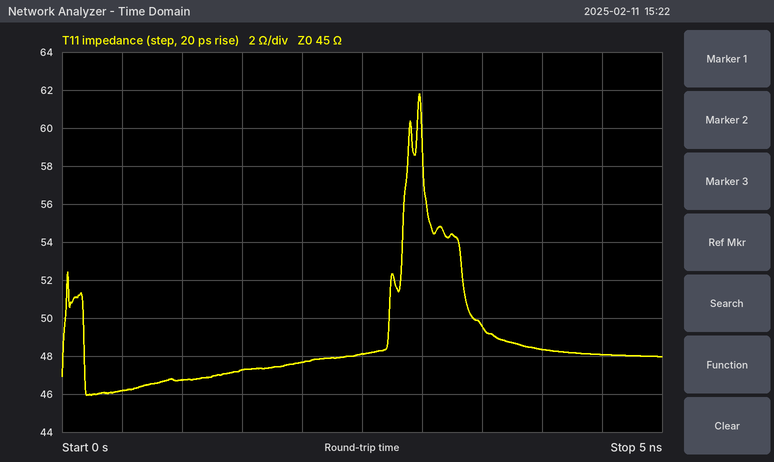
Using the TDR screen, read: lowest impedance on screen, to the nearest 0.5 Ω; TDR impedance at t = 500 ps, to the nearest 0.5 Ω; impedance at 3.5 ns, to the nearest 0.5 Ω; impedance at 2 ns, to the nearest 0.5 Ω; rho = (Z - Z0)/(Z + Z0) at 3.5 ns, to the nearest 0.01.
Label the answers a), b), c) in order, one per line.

a) 46.0 Ω
b) 46.0 Ω
c) 49.5 Ω
d) 47.5 Ω
e) +0.05
